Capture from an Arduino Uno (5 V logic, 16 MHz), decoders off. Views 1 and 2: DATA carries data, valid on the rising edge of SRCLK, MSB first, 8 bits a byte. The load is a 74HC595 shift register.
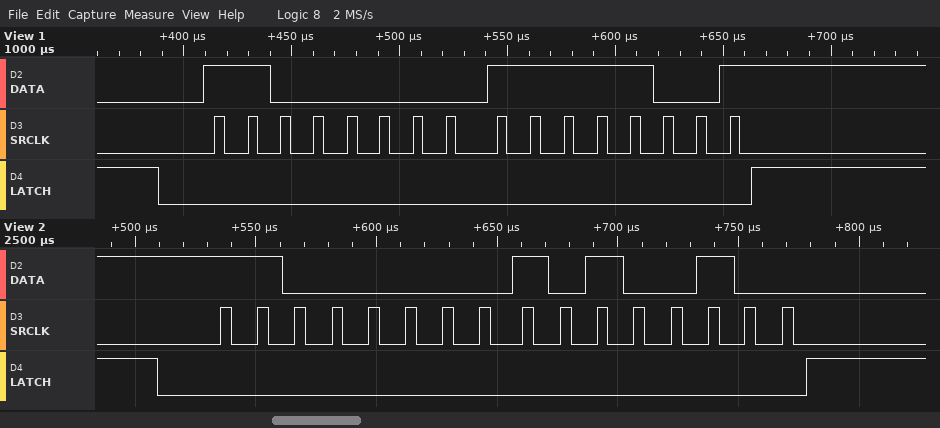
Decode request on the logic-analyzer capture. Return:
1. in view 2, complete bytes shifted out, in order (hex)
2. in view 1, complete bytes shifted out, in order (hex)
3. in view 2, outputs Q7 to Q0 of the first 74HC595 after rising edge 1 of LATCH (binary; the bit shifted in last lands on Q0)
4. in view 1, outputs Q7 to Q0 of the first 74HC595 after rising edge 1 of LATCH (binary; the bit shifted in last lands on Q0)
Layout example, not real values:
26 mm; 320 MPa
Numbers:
0xC0 0xA4; C0 F9; 10100100; 11111001
